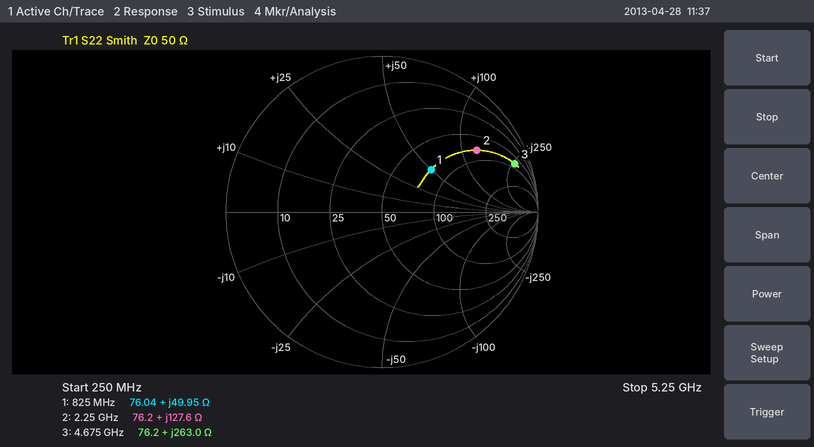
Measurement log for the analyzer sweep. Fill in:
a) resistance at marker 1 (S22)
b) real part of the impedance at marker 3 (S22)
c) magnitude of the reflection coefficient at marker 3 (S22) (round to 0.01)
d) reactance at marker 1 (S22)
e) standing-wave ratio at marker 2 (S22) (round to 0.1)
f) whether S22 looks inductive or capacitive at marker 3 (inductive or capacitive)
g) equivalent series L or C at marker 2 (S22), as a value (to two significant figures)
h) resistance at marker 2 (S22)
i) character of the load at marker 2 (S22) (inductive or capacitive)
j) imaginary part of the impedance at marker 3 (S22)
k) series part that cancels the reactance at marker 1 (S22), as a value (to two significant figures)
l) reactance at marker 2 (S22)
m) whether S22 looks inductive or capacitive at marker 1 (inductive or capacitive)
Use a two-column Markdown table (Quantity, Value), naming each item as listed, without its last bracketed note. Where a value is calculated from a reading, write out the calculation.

| Quantity | Value |
|---|---|
| resistance at marker 1 | 76.04 Ω |
| real part of the impedance at marker 3 | 76.2 Ω |
| magnitude of the reflection coefficient at marker 3 (S22) | 0.91 |
| reactance at marker 1 | +49.95 Ω |
| standing-wave ratio at marker 2 (S22) | 6.3 |
| whether S22 looks inductive or capacitive at marker 3 | inductive |
| equivalent series L or C at marker 2 (S22), as a value | L = 127.6 Ω/(2π × 2.25 GHz) ≈ 9.0 nH |
| resistance at marker 2 | 76.2 Ω |
| character of the load at marker 2 (S22) | inductive |
| imaginary part of the impedance at marker 3 | +263.0 Ω |
| series part that cancels the reactance at marker 1 (S22), as a value | C = 1/(2π × 825 MHz × 49.95 Ω) ≈ 3.9 pF |
| reactance at marker 2 | +127.6 Ω |
| whether S22 looks inductive or capacitive at marker 1 | inductive |
